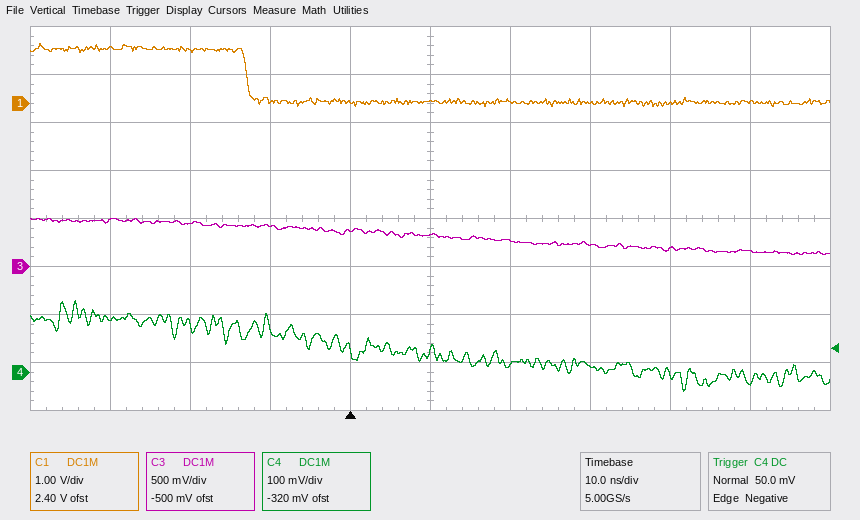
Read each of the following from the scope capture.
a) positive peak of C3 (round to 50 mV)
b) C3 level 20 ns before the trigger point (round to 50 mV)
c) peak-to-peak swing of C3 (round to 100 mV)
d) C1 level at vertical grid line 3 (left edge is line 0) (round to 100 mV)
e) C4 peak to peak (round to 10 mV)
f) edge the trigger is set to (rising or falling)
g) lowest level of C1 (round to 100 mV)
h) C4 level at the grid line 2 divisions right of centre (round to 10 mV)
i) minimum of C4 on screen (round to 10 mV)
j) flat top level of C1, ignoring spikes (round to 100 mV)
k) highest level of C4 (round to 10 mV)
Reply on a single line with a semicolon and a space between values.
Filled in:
500 mV; 450 mV; 400 mV; 100 mV; 190 mV; falling; -100 mV; 10 mV; -40 mV; 1.1 V; 150 mV
